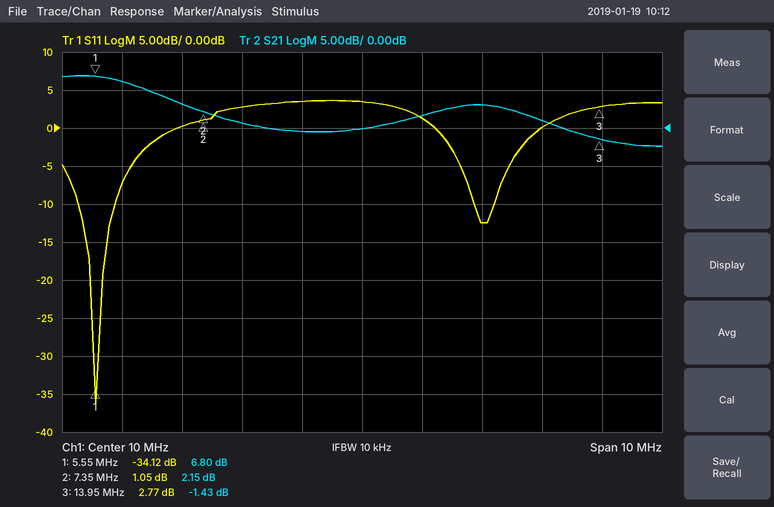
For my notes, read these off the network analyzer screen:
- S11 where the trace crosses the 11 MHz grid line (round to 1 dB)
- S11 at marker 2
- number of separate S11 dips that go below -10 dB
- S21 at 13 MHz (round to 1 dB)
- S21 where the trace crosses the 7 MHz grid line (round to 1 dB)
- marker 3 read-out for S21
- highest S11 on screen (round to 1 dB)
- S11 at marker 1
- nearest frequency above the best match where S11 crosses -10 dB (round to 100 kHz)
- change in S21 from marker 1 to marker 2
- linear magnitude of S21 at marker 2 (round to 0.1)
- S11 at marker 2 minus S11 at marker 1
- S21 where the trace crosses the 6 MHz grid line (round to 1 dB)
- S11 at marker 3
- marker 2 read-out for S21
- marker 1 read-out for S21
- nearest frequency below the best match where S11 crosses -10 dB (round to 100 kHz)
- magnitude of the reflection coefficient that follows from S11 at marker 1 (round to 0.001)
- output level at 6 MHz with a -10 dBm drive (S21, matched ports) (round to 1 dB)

1 dB
1.05 dB
2
1 dB
3 dB
-1.43 dB
4 dB
-34.12 dB
5.9 MHz
-4.65 dB
1.3
35.17 dB
6 dB
2.77 dB
2.15 dB
6.80 dB
5.3 MHz
0.020
-4 dBm
